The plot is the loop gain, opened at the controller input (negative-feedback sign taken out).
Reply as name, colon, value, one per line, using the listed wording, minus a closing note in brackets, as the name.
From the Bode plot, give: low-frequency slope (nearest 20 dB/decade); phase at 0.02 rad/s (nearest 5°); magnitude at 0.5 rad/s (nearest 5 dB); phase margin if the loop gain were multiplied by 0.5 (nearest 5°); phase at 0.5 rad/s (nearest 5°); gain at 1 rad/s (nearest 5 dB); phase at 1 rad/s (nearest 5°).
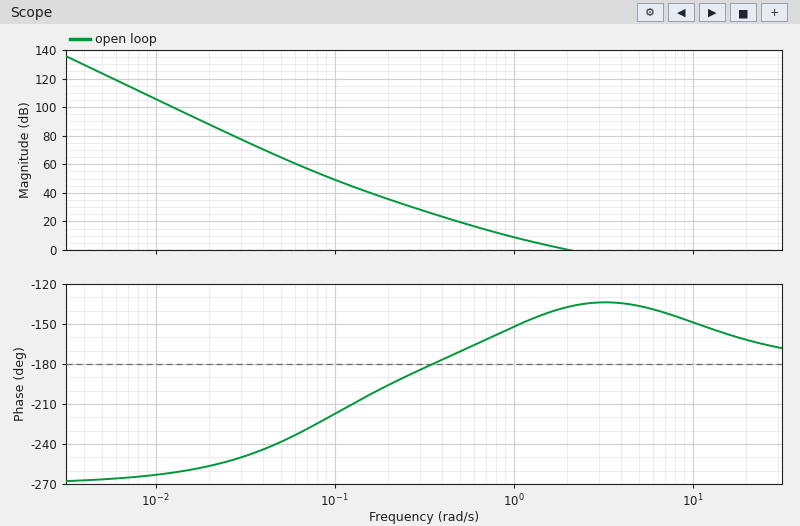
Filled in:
low-frequency slope: -60 dB/decade
phase at 0.02 rad/s: -255°
magnitude at 0.5 rad/s: 20 dB
phase margin if the loop gain were multiplied by 0.5: 35°
phase at 0.5 rad/s: -170°
gain at 1 rad/s: 10 dB
phase at 1 rad/s: -150°
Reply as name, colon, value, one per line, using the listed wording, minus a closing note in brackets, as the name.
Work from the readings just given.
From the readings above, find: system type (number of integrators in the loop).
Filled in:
system type: 3
